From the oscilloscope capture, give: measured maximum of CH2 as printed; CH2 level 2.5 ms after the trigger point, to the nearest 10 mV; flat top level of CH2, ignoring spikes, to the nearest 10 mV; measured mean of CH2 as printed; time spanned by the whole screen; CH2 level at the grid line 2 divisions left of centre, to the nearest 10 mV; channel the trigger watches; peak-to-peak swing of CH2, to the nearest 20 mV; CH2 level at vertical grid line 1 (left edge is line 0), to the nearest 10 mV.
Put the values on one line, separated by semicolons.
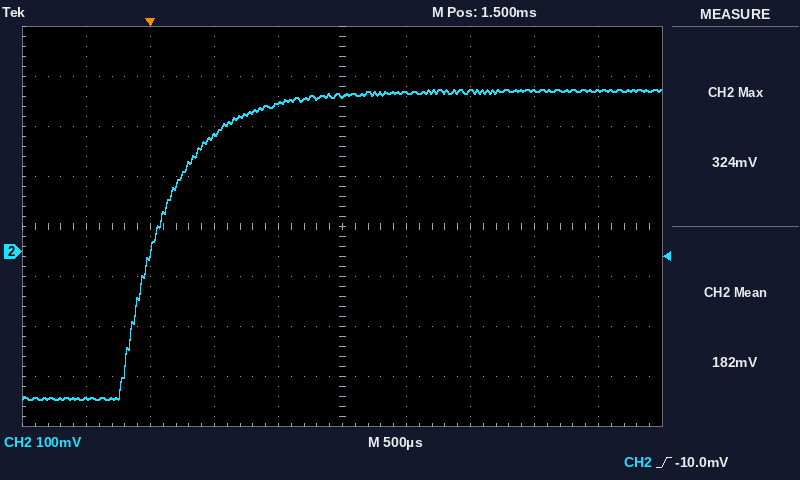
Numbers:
324 mV; 320 mV; 320 mV; 182 mV; 5 ms; 230 mV; CH2; 620 mV; -290 mV
